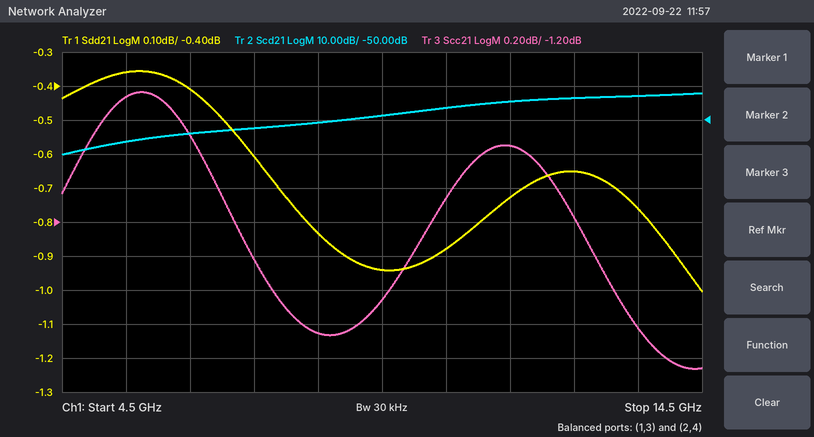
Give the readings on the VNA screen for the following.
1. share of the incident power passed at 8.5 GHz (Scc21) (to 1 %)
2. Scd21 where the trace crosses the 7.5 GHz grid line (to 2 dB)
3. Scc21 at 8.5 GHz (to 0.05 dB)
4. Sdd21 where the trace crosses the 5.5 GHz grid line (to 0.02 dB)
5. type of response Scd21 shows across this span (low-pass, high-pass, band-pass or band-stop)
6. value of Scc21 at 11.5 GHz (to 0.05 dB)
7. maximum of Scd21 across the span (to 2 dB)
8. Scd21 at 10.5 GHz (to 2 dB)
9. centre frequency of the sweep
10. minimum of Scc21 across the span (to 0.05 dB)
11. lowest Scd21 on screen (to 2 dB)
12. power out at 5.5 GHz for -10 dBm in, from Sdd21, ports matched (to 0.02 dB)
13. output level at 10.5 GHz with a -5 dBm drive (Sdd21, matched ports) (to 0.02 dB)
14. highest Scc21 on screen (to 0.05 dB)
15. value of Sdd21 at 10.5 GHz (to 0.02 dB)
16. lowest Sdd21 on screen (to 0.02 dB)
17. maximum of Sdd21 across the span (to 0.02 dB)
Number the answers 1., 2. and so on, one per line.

1. 65 %
2. -52 dB
3. -1.85 dB
4. -0.36 dB
5. high-pass
6. -0.75 dB
7. -42 dB
8. -46 dB
9. 9.5 GHz
10. -2.05 dB
11. -60 dB
12. -10.36 dBm
13. -5.88 dBm
14. -0.45 dB
15. -0.88 dB
16. -1.00 dB
17. -0.36 dB
